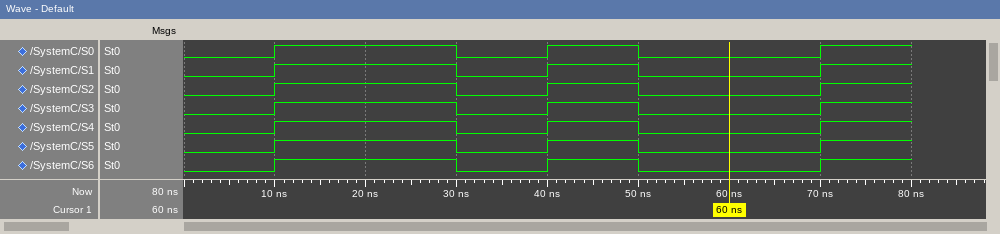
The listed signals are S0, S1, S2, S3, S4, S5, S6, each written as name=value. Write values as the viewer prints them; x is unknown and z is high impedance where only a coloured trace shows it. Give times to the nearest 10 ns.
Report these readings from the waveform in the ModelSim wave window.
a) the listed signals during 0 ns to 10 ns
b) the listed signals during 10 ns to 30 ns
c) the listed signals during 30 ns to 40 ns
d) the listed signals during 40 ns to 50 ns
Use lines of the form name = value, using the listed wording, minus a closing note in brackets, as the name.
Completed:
the listed signals during 0 ns to 10 ns = S0=0, S1=0, S2=0, S3=0, S4=0, S5=0, S6=0
the listed signals during 10 ns to 30 ns = S0=1, S1=1, S2=1, S3=1, S4=1, S5=1, S6=1
the listed signals during 30 ns to 40 ns = S0=0, S1=0, S2=0, S3=0, S4=0, S5=0, S6=0
the listed signals during 40 ns to 50 ns = S0=1, S1=1, S2=1, S3=1, S4=1, S5=1, S6=1
